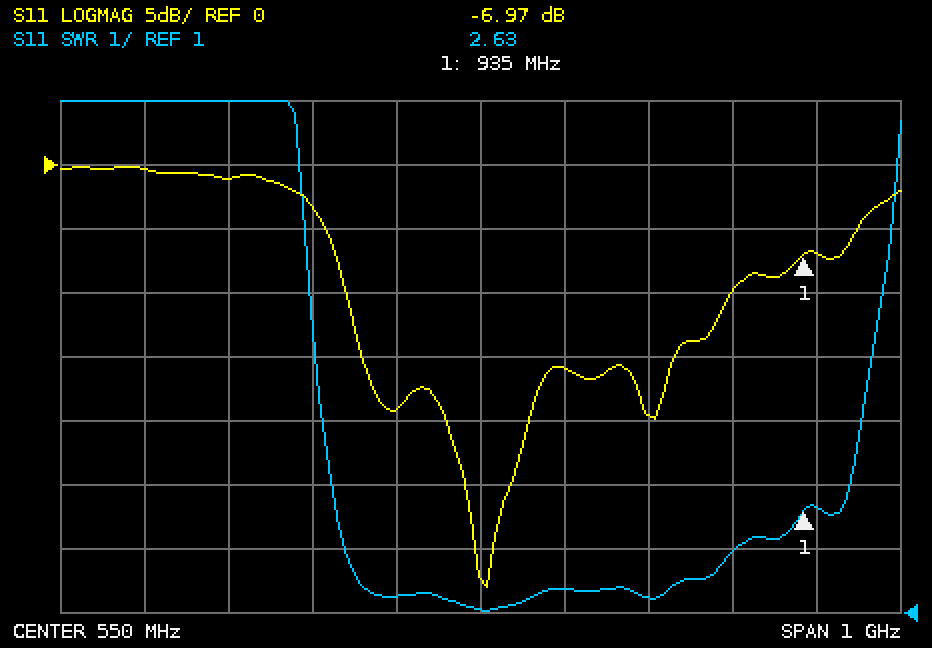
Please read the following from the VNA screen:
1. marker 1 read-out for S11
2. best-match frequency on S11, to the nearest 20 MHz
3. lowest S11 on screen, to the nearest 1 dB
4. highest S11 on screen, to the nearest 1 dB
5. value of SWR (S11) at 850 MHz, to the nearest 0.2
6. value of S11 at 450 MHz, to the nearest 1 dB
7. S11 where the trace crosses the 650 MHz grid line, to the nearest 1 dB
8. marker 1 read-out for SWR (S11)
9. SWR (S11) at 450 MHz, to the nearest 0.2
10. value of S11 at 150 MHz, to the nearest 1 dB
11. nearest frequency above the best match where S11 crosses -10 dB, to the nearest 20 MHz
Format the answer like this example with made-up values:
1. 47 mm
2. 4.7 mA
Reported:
1. -6.97 dB
2. 560 MHz
3. -33 dB
4. 0 dB
5. 2.0
6. -19 dB
7. -16 dB
8. 2.63
9. 1.2
10. 0 dB
11. 840 MHz
